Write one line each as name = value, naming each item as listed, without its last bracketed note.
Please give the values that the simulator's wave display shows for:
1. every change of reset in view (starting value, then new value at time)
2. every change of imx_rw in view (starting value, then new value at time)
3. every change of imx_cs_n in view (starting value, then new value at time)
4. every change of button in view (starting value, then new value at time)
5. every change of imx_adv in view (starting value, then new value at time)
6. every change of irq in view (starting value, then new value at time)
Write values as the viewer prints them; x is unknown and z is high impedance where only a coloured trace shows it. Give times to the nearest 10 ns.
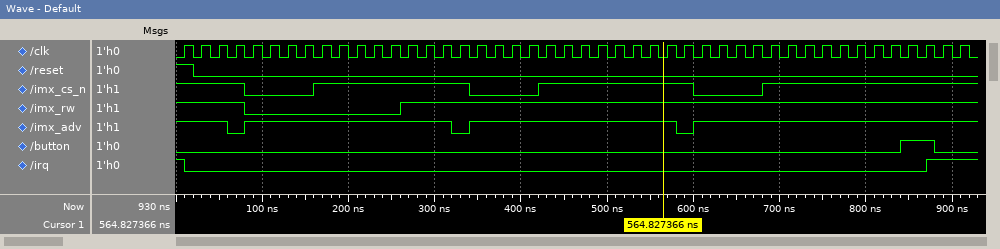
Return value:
every change of reset in view = 1, 0 at 20 ns
every change of imx_rw in view = 1, 0 at 80 ns, 1 at 260 ns
every change of imx_cs_n in view = 1, 0 at 80 ns, 1 at 160 ns, 0 at 340 ns, 1 at 420 ns, 0 at 600 ns, 1 at 680 ns
every change of button in view = 0, 1 at 840 ns, 0 at 880 ns
every change of imx_adv in view = 1, 0 at 60 ns, 1 at 80 ns, 0 at 320 ns, 1 at 340 ns, 0 at 580 ns, 1 at 600 ns
every change of irq in view = 1, 0 at 10 ns, 1 at 870 ns
